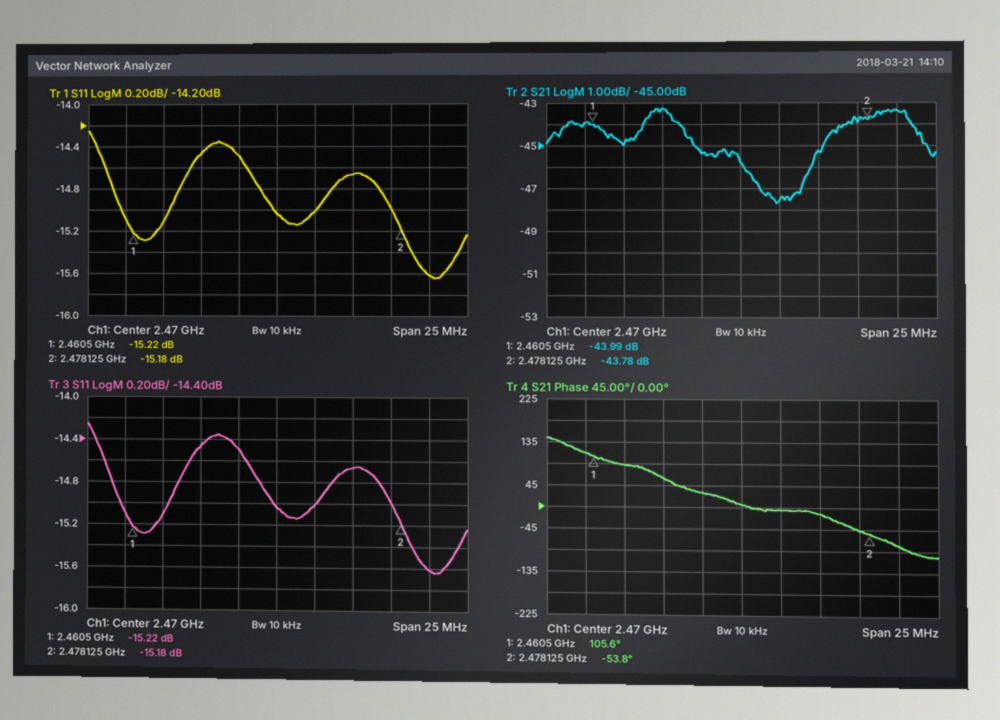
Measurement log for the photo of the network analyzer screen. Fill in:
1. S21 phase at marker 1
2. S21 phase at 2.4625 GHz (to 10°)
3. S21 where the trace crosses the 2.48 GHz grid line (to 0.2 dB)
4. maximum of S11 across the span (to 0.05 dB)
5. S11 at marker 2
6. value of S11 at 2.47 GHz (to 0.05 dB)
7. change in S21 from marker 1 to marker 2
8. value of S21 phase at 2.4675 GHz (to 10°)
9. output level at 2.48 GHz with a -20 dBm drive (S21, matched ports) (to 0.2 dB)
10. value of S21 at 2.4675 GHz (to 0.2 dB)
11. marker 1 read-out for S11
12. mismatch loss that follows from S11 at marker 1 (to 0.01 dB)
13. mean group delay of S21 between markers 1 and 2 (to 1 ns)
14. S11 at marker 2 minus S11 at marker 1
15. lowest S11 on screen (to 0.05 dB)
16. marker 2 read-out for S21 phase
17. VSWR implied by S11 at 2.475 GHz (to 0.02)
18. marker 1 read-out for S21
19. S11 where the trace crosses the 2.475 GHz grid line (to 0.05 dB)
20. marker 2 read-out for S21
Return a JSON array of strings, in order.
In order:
["105.6°", "90°", "-43.4 dB", "-14.25 dB", "-15.18 dB", "-15.05 dB", "0.21 dB", "30°", "-63.4 dBm", "-45.4 dB", "-15.22 dB", "0.13 dB", "25 ns", "0.04 dB", "-15.65 dB", "-53.8°", "1.46", "-43.99 dB", "-14.65 dB", "-43.78 dB"]
